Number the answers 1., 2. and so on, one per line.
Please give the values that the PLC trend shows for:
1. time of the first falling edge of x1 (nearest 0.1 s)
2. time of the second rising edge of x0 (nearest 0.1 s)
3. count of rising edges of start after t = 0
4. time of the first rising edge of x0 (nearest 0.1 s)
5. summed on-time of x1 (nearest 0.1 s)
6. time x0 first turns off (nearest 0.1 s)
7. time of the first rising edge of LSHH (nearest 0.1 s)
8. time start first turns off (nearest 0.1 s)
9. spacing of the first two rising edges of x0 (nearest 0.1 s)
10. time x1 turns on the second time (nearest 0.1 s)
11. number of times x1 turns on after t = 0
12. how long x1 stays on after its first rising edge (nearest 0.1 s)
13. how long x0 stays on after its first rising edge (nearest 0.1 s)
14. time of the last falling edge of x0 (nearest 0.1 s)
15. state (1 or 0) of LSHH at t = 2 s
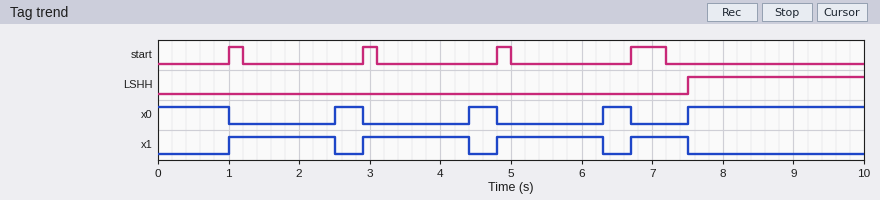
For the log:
1. 2.5 s
2. 4.4 s
3. 4
4. 2.5 s
5. 5.3 s
6. 1.0 s
7. 7.5 s
8. 1.2 s
9. 1.9 s
10. 2.9 s
11. 4
12. 1.5 s
13. 0.4 s
14. 6.7 s
15. 0
